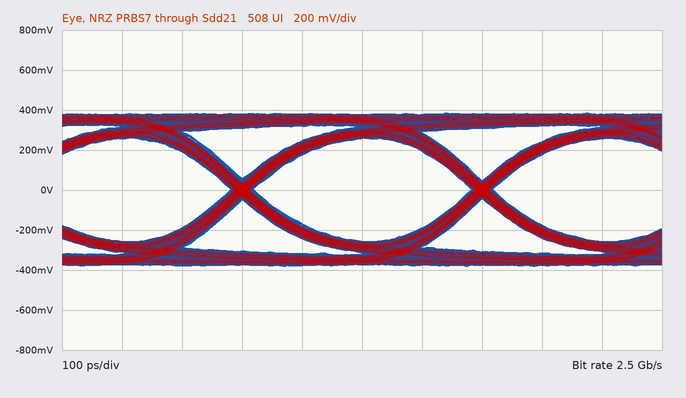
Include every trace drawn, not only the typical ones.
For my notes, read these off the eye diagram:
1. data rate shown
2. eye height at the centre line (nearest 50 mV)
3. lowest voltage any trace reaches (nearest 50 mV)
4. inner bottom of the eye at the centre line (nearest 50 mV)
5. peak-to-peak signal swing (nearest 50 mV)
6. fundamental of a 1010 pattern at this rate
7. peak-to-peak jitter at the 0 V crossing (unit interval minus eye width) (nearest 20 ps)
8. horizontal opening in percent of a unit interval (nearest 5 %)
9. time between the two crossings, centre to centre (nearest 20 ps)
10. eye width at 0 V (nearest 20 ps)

2.5 Gb/s
500 mV
-400 mV
-250 mV
750 mV
1.25 GHz
40 ps
90 %
400 ps
360 ps
